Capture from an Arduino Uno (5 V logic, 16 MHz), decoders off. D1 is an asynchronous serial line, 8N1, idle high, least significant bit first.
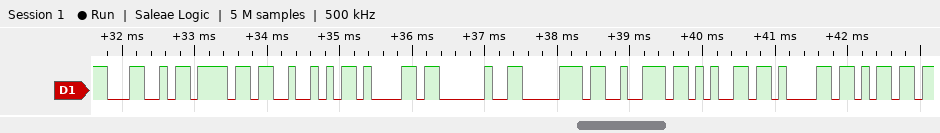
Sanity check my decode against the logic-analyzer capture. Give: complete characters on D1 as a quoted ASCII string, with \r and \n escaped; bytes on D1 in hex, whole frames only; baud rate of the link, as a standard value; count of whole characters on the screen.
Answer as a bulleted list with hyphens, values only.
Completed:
- "LoRa pream"
- 4C 6F 52 61 20 70 72 65 61 6D
- 9600 baud
- 10
